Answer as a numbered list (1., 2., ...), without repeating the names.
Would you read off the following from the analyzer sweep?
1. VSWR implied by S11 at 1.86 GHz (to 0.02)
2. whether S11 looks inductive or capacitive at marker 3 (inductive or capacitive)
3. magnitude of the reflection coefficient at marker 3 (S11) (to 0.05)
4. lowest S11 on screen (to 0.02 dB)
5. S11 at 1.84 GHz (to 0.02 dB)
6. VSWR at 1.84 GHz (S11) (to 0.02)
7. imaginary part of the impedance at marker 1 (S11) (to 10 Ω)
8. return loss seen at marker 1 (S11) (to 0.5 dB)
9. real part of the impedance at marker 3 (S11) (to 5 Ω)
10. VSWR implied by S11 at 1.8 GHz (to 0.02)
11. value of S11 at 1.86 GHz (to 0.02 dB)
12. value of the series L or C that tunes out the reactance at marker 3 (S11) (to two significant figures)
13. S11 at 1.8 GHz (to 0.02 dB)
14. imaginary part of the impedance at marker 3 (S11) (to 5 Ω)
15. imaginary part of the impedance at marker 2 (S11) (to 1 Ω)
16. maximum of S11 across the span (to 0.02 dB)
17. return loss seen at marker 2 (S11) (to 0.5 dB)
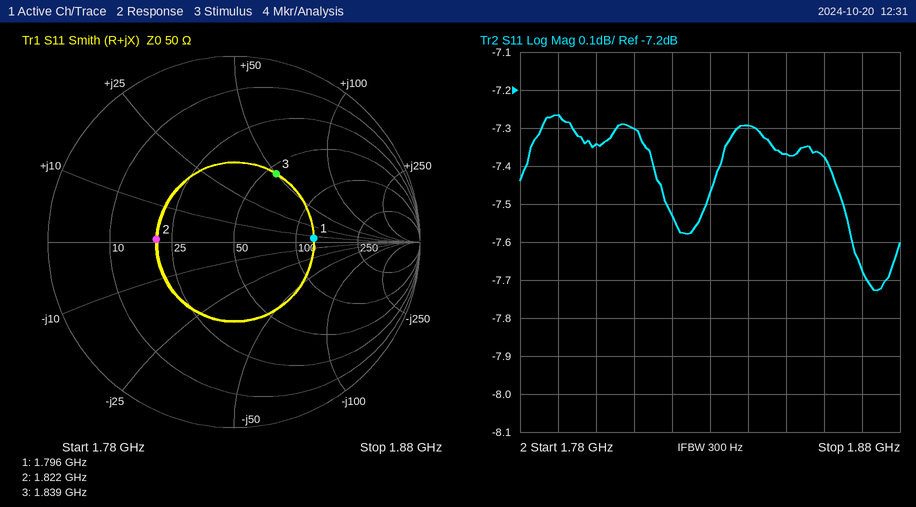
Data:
1. 2.50
2. inductive
3. 0.45
4. -7.72 dB
5. -7.30 dB
6. 2.52
7. +10 Ω
8. 7.5 dB
9. 55 Ω
10. 2.50
11. -7.38 dB
12. 1.7 pF
13. -7.34 dB
14. +50 Ω
15. +1 Ω
16. -7.26 dB
17. 7.5 dB
